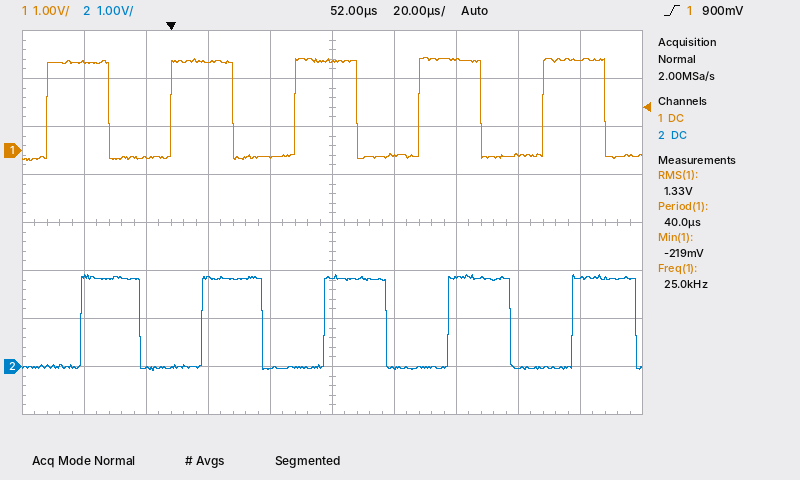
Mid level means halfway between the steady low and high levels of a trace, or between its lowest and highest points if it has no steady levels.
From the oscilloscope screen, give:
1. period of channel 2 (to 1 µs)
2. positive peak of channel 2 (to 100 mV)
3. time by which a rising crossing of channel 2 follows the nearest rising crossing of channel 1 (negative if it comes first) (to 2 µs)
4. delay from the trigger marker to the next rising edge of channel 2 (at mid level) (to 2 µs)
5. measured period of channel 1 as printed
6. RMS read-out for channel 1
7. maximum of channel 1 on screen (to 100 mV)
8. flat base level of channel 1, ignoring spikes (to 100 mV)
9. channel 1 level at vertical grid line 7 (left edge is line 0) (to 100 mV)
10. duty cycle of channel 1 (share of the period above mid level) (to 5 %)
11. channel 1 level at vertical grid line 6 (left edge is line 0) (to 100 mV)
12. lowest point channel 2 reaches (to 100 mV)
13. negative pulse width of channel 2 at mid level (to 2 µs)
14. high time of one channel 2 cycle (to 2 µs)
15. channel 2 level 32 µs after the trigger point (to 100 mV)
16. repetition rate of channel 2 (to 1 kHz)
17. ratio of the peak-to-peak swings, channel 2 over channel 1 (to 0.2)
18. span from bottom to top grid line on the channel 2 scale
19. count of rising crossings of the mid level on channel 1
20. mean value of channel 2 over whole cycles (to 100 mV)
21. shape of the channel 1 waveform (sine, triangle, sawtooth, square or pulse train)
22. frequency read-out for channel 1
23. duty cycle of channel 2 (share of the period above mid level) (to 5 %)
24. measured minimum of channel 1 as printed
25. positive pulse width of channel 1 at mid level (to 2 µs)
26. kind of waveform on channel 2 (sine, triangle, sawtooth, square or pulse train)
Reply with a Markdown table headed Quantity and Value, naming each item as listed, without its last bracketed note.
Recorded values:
| Quantity | Value |
|---|---|
| period of channel 2 | 40 µs |
| positive peak of channel 2 | 1.9 V |
| time by which a rising crossing of channel 2 follows the nearest rising crossing of channel 1 (negative if it comes first) | +10 µs |
| delay from the trigger marker to the next rising edge of channel 2 (at mid level) | 10 µs |
| measured period of channel 1 as printed | 40.0 µs |
| RMS read-out for channel 1 | 1.33 V |
| maximum of channel 1 on screen | 1.9 V |
| flat base level of channel 1, ignoring spikes | -100 mV |
| channel 1 level at vertical grid line 7 (left edge is line 0) | 1.9 V |
| duty cycle of channel 1 (share of the period above mid level) | 50 % |
| channel 1 level at vertical grid line 6 (left edge is line 0) | -100 mV |
| lowest point channel 2 reaches | -100 mV |
| negative pulse width of channel 2 at mid level | 20 µs |
| high time of one channel 2 cycle | 20 µs |
| channel 2 level 32 µs after the trigger point | 0.0 V |
| repetition rate of channel 2 | 25 kHz |
| ratio of the peak-to-peak swings, channel 2 over channel 1 | 1.0 |
| span from bottom to top grid line on the channel 2 scale | 8 V |
| count of rising crossings of the mid level on channel 1 | 5 |
| mean value of channel 2 over whole cycles | 900 mV |
| shape of the channel 1 waveform | square |
| frequency read-out for channel 1 | 25.0 kHz |
| duty cycle of channel 2 (share of the period above mid level) | 50 % |
| measured minimum of channel 1 as printed | -219 mV |
| positive pulse width of channel 1 at mid level | 20 µs |
| kind of waveform on channel 2 | square |
